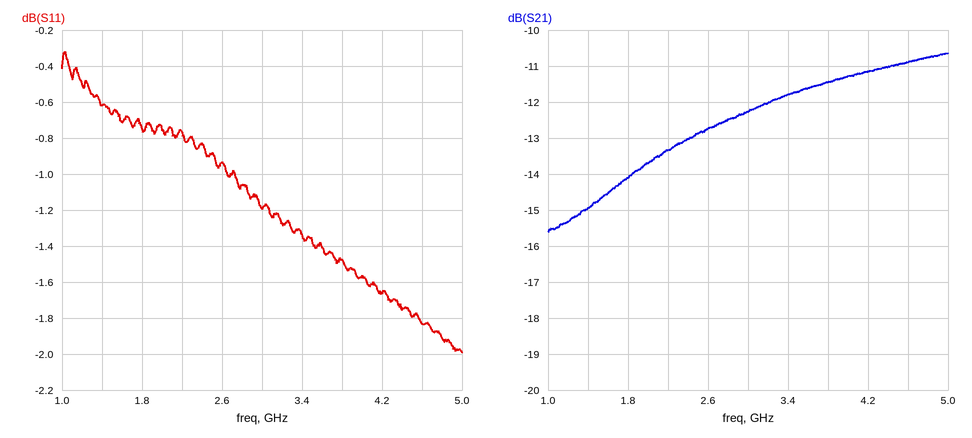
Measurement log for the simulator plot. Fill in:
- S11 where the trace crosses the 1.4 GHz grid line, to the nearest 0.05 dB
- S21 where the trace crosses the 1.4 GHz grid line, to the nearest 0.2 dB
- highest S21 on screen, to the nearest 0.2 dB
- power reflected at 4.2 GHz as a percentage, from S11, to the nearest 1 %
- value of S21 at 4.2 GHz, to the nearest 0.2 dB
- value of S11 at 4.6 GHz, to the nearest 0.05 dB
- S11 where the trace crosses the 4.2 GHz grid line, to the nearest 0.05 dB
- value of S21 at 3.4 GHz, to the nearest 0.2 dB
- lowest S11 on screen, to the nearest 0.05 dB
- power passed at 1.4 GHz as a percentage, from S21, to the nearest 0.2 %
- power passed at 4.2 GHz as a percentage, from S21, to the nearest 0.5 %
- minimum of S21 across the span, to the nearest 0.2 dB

-0.60 dB
-15.0 dB
-10.6 dB
68 %
-11.2 dB
-1.85 dB
-1.65 dB
-11.8 dB
-2.00 dB
3.2 %
7.5 %
-15.6 dB
